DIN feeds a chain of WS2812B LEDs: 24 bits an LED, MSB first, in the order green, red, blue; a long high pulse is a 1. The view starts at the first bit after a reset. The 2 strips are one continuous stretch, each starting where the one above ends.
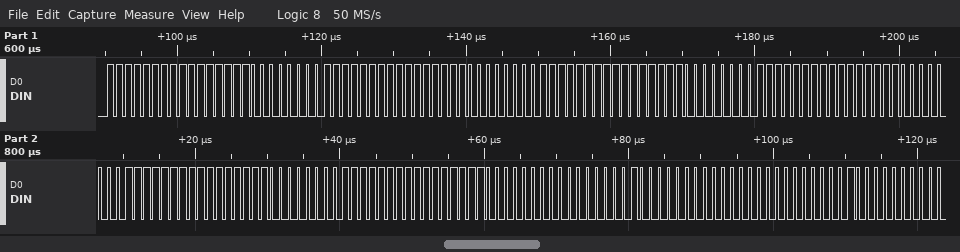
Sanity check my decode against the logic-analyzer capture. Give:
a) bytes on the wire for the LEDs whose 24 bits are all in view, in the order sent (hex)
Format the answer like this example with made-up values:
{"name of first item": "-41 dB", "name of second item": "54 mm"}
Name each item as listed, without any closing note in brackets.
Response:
{"bytes on the wire for the LEDs whose 24 bits are all in view, in the order sent": "FF FF 00 FF FF 00 FF FF 00 FF FF 00 FF FF 00 FF FF 00 00 80 00"}
